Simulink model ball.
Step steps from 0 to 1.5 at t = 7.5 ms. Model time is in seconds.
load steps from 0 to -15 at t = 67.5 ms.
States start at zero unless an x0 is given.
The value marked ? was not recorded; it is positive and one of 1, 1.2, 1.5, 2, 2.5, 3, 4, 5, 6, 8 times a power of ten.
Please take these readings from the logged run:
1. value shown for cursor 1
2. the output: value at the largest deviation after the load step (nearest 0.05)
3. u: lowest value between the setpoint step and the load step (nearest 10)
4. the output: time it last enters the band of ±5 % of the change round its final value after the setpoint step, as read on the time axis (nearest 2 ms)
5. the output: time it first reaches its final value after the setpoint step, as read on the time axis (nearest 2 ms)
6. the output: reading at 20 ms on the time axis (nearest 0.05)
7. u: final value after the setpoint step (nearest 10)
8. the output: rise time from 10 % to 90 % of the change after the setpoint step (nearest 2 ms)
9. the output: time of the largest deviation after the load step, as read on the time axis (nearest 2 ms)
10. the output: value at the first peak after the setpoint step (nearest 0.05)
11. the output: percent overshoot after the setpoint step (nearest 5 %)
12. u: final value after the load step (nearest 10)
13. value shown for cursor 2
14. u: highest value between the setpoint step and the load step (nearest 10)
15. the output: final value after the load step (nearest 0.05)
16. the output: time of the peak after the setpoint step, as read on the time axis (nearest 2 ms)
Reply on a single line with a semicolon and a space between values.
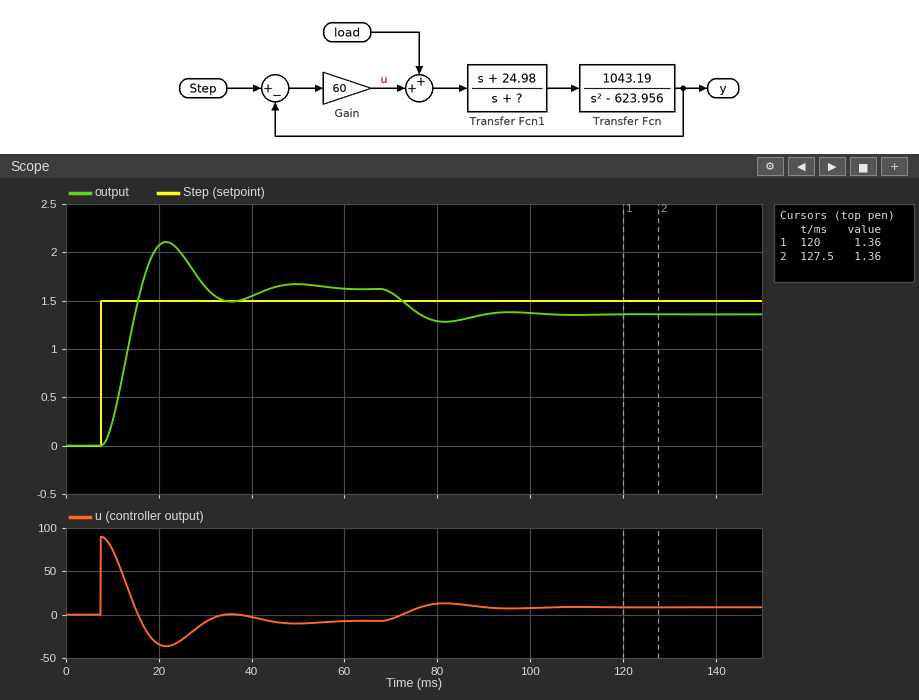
1.36; 1.30; -40; 40 ms; 16 ms; 2.05; -10; 6 ms; 82 ms; 2.10; 30 %; 10; 1.36; 90; 1.35; 22 ms
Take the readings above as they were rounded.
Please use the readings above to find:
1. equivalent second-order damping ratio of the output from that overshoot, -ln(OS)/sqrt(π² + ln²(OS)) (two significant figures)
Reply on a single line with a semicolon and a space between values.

0.36
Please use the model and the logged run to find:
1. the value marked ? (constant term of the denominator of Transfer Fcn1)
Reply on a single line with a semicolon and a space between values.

200
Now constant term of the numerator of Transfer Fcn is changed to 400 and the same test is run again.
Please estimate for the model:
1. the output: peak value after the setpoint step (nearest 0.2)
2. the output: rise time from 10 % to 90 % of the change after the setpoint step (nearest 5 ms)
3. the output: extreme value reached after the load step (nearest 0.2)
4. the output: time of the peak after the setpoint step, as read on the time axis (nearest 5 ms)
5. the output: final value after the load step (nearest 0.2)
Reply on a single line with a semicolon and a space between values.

2.0; 15 ms; 1.6; 35 ms; 1.6
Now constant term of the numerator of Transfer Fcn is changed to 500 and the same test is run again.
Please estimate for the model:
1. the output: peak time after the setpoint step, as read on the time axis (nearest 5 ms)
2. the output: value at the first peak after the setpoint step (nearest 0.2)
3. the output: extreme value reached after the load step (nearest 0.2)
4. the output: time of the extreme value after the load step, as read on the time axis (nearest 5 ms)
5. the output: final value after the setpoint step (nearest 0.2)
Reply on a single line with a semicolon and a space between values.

30 ms; 2.0; 1.4; 90 ms; 1.8
